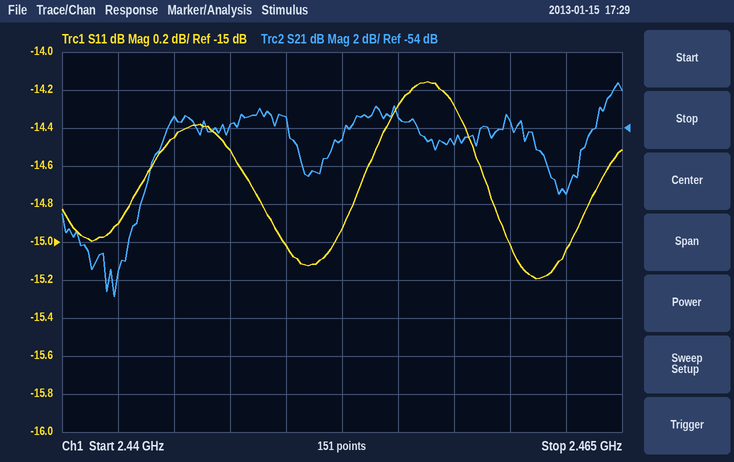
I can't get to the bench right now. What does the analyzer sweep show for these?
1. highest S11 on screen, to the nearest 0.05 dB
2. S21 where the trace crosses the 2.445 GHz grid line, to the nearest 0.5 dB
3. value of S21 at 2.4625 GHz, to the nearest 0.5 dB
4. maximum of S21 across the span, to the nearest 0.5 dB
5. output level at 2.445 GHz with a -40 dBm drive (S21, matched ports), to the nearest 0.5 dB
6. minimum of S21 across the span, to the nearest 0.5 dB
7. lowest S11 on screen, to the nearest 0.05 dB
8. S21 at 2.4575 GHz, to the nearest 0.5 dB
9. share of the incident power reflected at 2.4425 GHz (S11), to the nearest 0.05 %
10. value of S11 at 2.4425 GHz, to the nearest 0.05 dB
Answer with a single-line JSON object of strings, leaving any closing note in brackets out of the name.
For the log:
{"highest S11 on screen, to the nearest 0.05 dB": "-14.15 dB", "S21 where the trace crosses the 2.445 GHz grid line, to the nearest 0.5 dB": "-53.5 dB", "value of S21 at 2.4625 GHz, to the nearest 0.5 dB": "-57.5 dB", "maximum of S21 across the span, to the nearest 0.5 dB": "-51.5 dB", "output level at 2.445 GHz with a -40 dBm drive (S21, matched ports), to the nearest 0.5 dB": "-93.5 dBm", "minimum of S21 across the span, to the nearest 0.5 dB": "-63.0 dB", "lowest S11 on screen, to the nearest 0.05 dB": "-15.20 dB", "S21 at 2.4575 GHz, to the nearest 0.5 dB": "-55.0 dB", "share of the incident power reflected at 2.4425 GHz (S11), to the nearest 0.05 %": "3.25 %", "value of S11 at 2.4425 GHz, to the nearest 0.05 dB": "-14.90 dB"}
